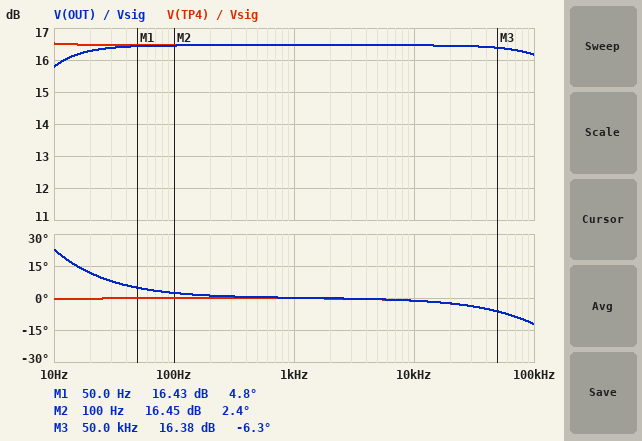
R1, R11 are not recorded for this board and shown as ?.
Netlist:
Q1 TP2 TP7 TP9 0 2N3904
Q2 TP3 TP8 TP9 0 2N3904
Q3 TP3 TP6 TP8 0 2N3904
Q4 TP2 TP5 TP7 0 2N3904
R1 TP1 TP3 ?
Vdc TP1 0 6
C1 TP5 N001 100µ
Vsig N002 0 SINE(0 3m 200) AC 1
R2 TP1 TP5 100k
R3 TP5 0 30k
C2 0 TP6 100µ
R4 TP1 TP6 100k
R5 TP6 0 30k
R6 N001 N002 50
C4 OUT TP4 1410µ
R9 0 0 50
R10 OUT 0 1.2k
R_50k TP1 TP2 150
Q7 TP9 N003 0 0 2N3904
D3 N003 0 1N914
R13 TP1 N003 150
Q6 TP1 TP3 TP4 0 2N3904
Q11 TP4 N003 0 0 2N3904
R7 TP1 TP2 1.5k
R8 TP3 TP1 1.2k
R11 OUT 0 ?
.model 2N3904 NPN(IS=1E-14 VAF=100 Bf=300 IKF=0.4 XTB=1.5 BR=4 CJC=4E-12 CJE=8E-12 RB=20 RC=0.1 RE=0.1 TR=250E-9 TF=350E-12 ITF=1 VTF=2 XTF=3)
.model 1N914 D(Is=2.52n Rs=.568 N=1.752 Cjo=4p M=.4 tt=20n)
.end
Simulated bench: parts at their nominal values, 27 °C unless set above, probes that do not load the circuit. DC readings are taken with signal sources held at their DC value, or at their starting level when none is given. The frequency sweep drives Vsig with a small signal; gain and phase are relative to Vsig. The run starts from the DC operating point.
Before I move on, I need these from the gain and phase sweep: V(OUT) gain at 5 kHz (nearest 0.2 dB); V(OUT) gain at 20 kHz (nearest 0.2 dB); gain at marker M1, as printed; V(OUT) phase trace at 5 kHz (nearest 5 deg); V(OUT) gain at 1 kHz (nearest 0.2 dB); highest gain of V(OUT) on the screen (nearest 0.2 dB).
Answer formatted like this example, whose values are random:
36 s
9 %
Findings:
16.4 dB
16.4 dB
16.43 dB
0 deg
16.4 dB
16.4 dB
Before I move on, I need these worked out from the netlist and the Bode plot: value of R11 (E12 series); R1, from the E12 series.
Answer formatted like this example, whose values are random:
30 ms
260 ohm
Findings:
27 Ω
100 Ω
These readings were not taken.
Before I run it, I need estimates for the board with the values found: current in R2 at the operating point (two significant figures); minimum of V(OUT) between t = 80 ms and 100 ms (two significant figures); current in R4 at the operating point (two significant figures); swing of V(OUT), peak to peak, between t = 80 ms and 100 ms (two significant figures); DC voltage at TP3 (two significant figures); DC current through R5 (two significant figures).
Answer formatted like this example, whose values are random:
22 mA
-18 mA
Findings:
46 µA
-20 mV
46 µA
40 mV
4.6 V
46 µA
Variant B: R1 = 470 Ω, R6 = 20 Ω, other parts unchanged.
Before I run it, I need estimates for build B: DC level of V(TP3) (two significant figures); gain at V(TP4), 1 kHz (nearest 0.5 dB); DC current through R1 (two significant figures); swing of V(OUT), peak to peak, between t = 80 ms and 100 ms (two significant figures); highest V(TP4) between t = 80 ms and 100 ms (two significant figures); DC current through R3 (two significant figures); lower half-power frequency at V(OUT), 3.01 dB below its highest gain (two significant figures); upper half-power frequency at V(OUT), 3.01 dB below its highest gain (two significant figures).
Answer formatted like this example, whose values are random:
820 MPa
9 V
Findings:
1.1 V
27.0 dB
10 mA
130 mV
420 mV
46 µA
4.0 Hz
390 kHz
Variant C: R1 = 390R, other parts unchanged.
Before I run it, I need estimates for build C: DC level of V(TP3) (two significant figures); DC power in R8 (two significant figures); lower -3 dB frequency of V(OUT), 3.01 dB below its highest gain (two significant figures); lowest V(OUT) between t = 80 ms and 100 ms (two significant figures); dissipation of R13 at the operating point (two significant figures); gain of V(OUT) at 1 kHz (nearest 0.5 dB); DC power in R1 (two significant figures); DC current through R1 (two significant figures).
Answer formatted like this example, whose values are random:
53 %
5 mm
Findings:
1.7 V
15 mW
4.0 Hz
-59 mV
180 mW
26.0 dB
47 mW
11 mA
